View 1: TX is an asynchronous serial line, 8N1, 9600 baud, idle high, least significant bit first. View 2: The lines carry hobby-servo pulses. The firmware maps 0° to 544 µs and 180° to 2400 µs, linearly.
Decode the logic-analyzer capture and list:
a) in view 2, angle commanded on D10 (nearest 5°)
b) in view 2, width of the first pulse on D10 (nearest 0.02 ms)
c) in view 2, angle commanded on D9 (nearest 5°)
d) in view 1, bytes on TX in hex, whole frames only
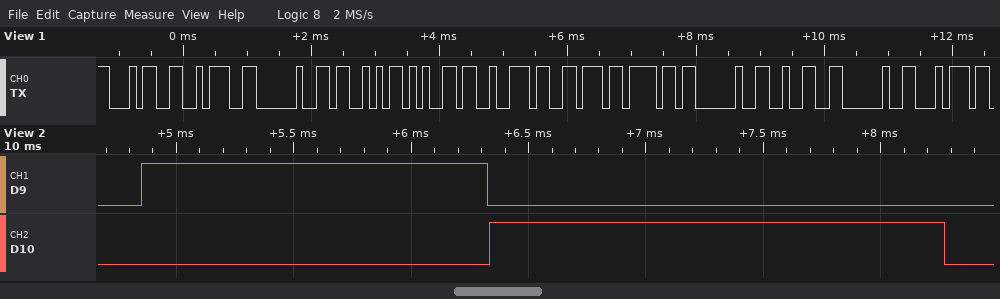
135°
1.94 ms
90°
34 3A 20 53 65 72 76 6F 20 32 20 74
